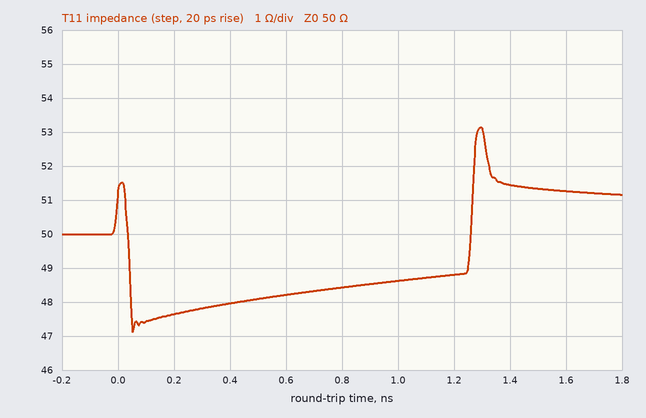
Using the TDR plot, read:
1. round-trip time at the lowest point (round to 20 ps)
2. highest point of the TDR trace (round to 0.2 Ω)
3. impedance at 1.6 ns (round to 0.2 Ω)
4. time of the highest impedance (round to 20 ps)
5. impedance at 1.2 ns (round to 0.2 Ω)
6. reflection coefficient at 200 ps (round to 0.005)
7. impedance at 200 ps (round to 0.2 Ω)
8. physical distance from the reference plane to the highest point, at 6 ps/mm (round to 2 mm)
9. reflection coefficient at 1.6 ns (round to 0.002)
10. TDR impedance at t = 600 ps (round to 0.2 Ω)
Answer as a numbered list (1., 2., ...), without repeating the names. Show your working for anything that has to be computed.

1. 60 ps
2. 53.2 Ω
3. 51.2 Ω
4. 1.30 ns
5. 48.8 Ω
6. (47.6 − 50)/(47.6 + 50) ≈ -0.025
7. 47.6 Ω
8. 1.30 ns / 2 / 6 ps/mm ≈ 108 mm
9. (51.2 − 50)/(51.2 + 50) ≈ +0.012
10. 48.2 Ω
